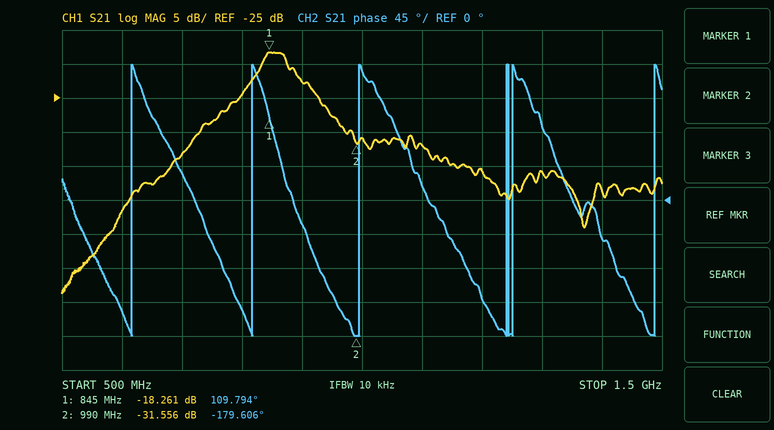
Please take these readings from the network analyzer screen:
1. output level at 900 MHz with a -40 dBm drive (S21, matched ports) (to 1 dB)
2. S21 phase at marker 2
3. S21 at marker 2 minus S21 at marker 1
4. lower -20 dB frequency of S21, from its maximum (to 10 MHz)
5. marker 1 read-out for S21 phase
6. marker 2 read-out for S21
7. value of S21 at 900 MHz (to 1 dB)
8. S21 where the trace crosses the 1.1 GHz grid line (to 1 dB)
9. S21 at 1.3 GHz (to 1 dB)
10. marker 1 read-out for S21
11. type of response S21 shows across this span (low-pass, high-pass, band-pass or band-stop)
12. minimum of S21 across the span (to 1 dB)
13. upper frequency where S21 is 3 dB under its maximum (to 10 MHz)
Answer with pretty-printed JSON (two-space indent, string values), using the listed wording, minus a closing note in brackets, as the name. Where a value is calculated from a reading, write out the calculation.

{
  "output level at 900 MHz with a -40 dBm drive (S21, matched ports)": "-40 dBm + (-23 dB) = -63 dBm",
  "S21 phase at marker 2": "-179.606°",
  "S21 at marker 2 minus S21 at marker 1": "-31.556 − (-18.261) = -13.295 dB",
  "lower -20 dB frequency of S21, from its maximum": "630 MHz",
  "marker 1 read-out for S21 phase": "109.794°",
  "marker 2 read-out for S21": "-31.556 dB",
  "value of S21 at 900 MHz": "-23 dB",
  "S21 where the trace crosses the 1.1 GHz grid line": "-32 dB",
  "S21 at 1.3 GHz": "-36 dB",
  "marker 1 read-out for S21": "-18.261 dB",
  "type of response S21 shows across this span": "band-pass",
  "minimum of S21 across the span": "-54 dB",
  "upper frequency where S21 is 3 dB under its maximum": "890 MHz"
}
